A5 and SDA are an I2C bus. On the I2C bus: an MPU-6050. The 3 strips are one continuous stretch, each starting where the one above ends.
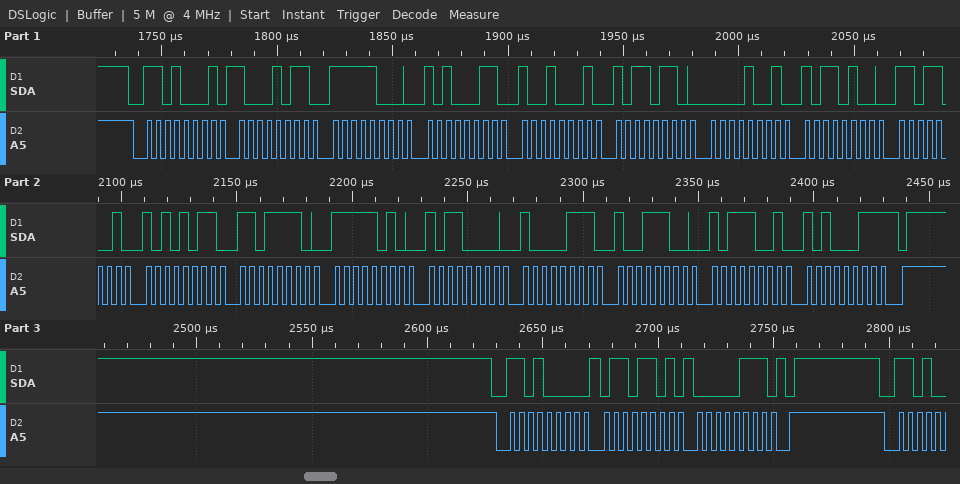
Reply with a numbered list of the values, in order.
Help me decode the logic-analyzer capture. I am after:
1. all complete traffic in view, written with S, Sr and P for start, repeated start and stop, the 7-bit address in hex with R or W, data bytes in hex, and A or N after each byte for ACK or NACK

1. S 68R A 8B A F8 A A3 A 91 A B6 A 09 A B4 A D9 A AB A DE A FA A B0 A 87 A 9C A B9 A A3 N P S 68W A 6D A 07 A P
